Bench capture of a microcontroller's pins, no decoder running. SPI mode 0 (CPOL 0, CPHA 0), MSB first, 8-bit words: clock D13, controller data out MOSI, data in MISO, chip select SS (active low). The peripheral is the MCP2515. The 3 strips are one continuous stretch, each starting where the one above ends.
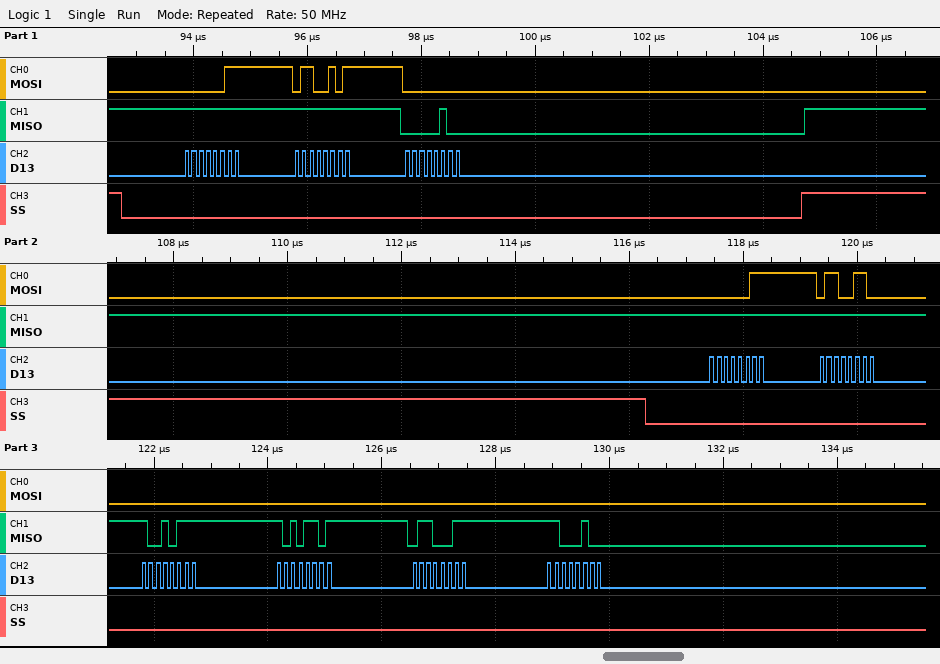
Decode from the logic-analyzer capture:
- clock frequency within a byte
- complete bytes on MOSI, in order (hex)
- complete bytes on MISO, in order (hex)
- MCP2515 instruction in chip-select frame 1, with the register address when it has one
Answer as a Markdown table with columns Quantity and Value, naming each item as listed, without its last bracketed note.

| Quantity | Value |
|---|---|
| clock frequency within a byte | 8 MHz |
| complete bytes on MOSI, in order | 03 65 00 03 66 00 00 00 00 |
| complete bytes on MISO, in order | FF FF 04 FF FF 97 AD 63 C4 |
| MCP2515 instruction in chip-select frame 1, with the register address when it has one | READ 0x65 |
